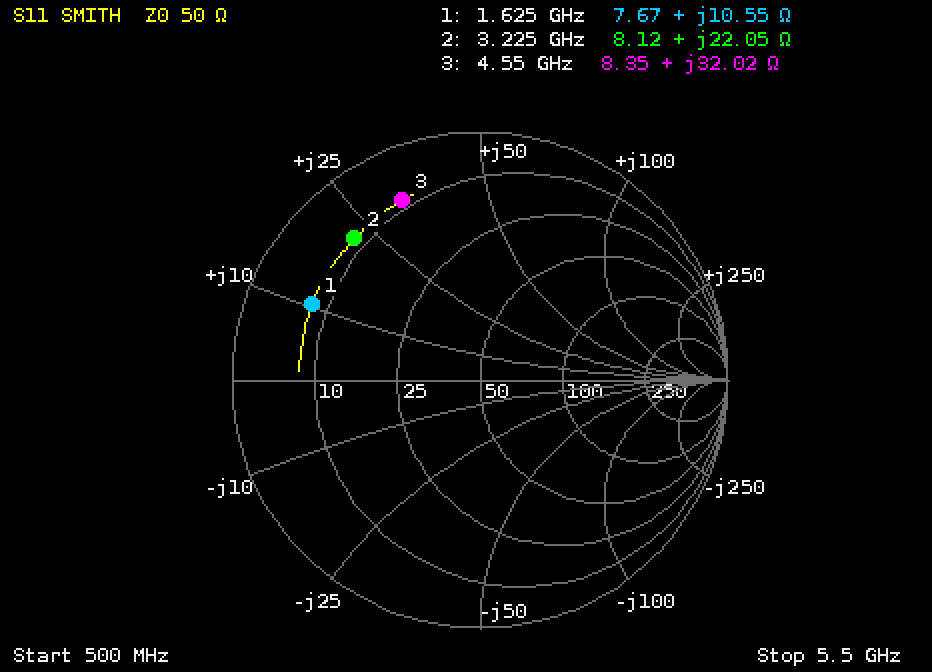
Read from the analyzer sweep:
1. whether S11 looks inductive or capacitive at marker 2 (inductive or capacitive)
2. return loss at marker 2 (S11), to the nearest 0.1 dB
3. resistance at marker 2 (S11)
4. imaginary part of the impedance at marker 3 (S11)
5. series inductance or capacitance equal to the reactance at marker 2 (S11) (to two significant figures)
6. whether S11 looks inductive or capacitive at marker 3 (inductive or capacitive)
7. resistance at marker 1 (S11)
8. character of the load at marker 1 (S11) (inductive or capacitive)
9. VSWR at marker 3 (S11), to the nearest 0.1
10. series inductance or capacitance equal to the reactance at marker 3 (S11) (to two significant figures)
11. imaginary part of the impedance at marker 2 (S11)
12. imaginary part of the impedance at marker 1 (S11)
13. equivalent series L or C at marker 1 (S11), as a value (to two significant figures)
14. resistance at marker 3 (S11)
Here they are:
inductive
2.4 dB
8.12 Ω
+32.02 Ω
1.1 nH
inductive
7.67 Ω
inductive
8.5
1.1 nH
+22.05 Ω
+10.55 Ω
1.0 nH
8.35 Ω
